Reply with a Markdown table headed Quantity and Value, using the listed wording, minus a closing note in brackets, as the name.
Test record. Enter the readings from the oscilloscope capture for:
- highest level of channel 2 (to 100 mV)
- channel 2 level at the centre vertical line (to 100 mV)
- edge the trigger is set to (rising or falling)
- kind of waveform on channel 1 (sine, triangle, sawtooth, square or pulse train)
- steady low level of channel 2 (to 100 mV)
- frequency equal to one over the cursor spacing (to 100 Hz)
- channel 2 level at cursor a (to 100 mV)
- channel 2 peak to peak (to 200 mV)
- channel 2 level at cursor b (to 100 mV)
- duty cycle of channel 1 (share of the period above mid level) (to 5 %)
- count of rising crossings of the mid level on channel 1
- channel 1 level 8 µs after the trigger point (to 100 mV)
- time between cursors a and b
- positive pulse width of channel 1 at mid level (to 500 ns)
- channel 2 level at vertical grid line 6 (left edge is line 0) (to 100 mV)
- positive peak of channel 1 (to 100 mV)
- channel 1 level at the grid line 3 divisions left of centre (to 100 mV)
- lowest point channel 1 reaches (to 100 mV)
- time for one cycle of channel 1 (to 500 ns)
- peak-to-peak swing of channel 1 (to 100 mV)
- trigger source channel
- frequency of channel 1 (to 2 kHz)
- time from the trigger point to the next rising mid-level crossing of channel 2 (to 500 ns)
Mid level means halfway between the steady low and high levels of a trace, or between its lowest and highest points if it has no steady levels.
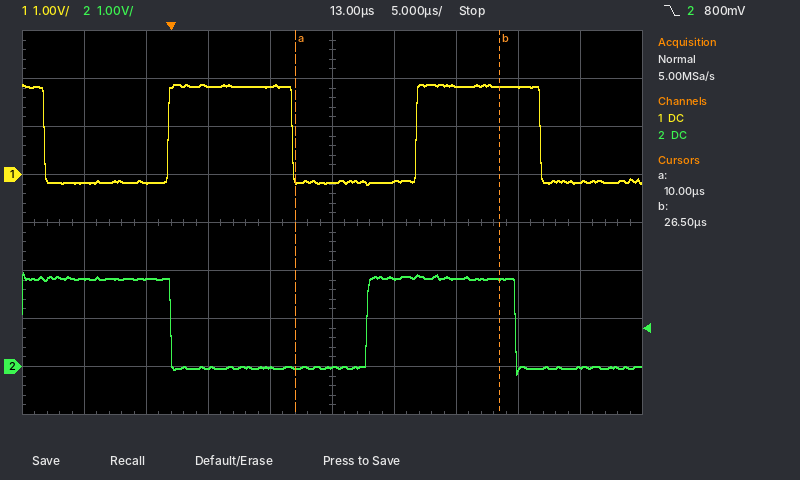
| Quantity | Value |
|---|---|
| highest level of channel 2 | 2.0 V |
| channel 2 level at the centre vertical line | 0.0 V |
| edge the trigger is set to | falling |
| kind of waveform on channel 1 | square |
| steady low level of channel 2 | 0.0 V |
| frequency equal to one over the cursor spacing | 60.6 kHz |
| channel 2 level at cursor a | 0.0 V |
| channel 2 peak to peak | 2.2 V |
| channel 2 level at cursor b | 1.8 V |
| duty cycle of channel 1 (share of the period above mid level) | 50 % |
| count of rising crossings of the mid level on channel 1 | 2 |
| channel 1 level 8 µs after the trigger point | 1.8 V |
| time between cursors a and b | 16.5 µs |
| positive pulse width of channel 1 at mid level | 10.0 µs |
| channel 2 level at vertical grid line 6 (left edge is line 0) | 1.8 V |
| positive peak of channel 1 | 1.9 V |
| channel 1 level at the grid line 3 divisions left of centre | -200 mV |
| lowest point channel 1 reaches | -200 mV |
| time for one cycle of channel 1 | 20.0 µs |
| peak-to-peak swing of channel 1 | 2.1 V |
| trigger source channel | channel 2 |
| frequency of channel 1 | 50 kHz |
| time from the trigger point to the next rising mid-level crossing of channel 2 | 16.0 µs |
